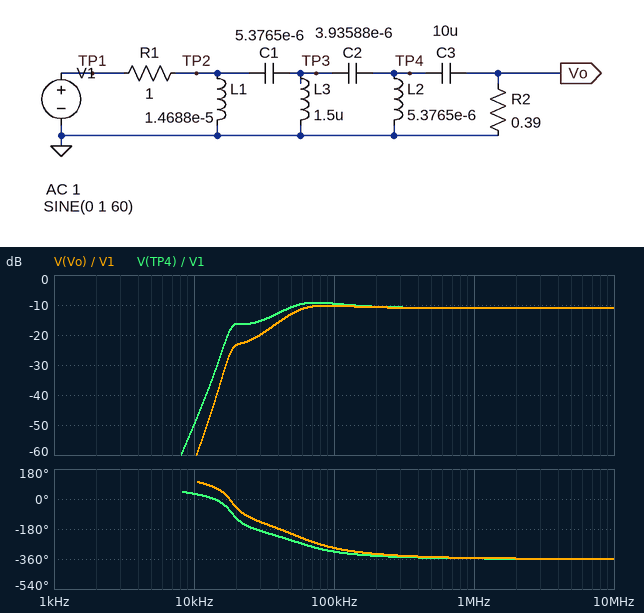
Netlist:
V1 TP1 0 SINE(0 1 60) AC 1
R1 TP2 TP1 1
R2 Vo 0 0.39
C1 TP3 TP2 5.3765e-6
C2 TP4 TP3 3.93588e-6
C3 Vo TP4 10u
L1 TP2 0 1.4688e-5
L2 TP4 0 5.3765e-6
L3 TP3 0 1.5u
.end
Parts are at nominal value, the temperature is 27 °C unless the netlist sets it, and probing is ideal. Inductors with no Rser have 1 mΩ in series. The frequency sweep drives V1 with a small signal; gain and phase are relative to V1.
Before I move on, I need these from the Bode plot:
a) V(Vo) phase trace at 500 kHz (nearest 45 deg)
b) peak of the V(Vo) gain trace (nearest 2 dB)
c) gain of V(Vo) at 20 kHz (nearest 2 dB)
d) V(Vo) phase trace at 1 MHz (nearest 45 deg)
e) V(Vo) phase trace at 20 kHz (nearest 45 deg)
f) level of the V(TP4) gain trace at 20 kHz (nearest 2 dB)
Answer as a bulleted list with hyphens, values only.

- -360 deg
- -10 dB
- -24 dB
- -360 deg
- -45 deg
- -16 dB
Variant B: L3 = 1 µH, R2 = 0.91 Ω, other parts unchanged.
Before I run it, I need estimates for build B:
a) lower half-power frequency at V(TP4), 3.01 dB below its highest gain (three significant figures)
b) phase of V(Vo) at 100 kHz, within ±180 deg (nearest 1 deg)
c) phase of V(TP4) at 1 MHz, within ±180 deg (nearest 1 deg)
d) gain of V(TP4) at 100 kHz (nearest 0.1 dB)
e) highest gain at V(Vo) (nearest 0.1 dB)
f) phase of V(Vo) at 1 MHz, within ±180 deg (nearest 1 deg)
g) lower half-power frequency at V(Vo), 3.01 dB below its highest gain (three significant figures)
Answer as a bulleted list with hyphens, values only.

- 60.5 kHz
- 80 deg
- 7 deg
- -7.5 dB
- -6.4 dB
- 8 deg
- 63.9 kHz
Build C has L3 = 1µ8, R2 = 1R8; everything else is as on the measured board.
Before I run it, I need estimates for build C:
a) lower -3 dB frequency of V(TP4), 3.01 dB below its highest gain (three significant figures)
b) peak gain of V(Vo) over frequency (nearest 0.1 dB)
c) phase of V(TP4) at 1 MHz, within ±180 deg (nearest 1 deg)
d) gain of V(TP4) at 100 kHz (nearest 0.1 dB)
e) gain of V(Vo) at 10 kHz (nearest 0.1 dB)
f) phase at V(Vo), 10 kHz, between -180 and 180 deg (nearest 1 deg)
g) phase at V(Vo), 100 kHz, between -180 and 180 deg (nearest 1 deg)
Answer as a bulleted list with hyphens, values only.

- 27.3 kHz
- -3.8 dB
- 6 deg
- -4.6 dB
- -52.1 dB
- 70 deg
- 63 deg
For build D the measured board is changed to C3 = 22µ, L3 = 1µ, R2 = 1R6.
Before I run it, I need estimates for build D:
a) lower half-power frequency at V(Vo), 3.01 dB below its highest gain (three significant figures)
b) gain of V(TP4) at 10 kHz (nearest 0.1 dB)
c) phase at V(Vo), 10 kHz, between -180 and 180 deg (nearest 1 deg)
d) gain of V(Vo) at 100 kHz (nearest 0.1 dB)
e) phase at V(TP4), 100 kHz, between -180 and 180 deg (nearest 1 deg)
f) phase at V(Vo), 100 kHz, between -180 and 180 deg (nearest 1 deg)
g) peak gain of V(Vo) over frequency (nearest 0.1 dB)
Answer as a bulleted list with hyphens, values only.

- 82.0 kHz
- -55.2 dB
- 48 deg
- -6.6 dB
- 74 deg
- 77 deg
- -4.2 dB
